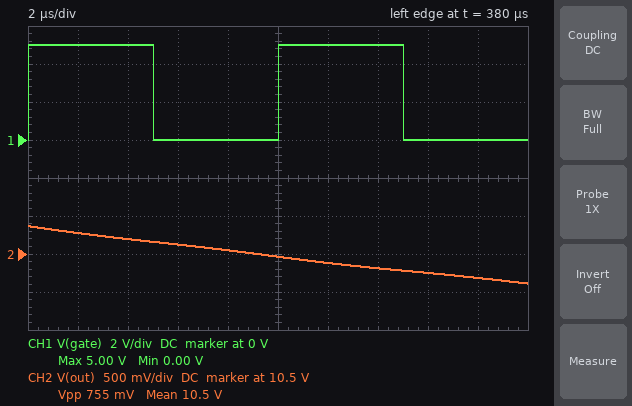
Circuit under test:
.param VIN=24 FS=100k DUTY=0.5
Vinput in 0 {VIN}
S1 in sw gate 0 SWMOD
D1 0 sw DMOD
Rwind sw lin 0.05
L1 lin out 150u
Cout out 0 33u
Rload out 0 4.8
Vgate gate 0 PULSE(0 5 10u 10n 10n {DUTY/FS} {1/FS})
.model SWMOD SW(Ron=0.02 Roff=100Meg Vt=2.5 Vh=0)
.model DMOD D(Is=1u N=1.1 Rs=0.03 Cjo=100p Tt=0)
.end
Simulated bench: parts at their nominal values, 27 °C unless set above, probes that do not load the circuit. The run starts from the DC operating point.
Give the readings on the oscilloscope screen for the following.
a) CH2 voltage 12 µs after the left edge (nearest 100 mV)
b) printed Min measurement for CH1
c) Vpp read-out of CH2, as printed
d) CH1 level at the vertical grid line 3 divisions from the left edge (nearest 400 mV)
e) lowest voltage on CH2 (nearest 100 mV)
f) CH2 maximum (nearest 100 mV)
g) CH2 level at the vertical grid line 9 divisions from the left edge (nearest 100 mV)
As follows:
10.4 V
0.00 V
755 mV
0 V
10.1 V
10.9 V
10.2 V
